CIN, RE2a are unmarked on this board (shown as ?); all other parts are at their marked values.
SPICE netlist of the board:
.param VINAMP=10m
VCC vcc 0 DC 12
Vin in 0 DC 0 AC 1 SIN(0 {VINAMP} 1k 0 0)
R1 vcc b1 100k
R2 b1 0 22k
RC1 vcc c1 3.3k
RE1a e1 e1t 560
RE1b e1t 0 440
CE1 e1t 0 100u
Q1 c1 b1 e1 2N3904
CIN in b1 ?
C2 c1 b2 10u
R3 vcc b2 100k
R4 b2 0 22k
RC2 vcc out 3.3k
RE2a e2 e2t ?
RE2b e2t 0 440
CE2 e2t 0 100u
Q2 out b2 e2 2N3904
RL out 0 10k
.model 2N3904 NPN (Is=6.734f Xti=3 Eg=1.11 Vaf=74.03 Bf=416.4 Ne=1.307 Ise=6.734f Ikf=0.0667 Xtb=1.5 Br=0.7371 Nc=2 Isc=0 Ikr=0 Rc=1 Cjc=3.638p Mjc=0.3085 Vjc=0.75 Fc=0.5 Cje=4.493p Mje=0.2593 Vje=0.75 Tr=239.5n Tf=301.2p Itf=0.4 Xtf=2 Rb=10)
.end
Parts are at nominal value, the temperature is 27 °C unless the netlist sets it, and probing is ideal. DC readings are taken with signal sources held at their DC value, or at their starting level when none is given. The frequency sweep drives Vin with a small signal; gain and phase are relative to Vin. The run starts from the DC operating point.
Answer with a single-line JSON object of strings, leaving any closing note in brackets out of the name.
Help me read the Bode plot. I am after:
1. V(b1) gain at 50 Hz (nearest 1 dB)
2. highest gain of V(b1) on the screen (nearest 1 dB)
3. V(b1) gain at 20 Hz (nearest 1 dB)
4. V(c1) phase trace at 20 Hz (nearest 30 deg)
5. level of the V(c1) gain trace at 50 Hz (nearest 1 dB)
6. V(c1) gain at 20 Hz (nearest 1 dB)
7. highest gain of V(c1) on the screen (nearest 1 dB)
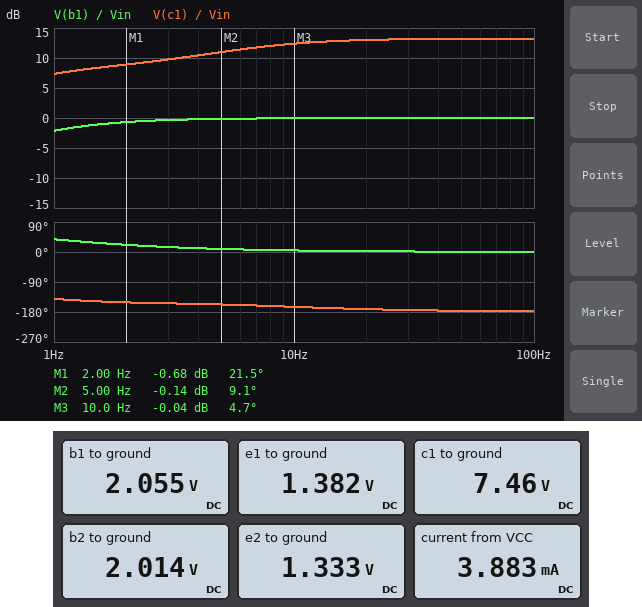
{"V(b1) gain at 50 Hz": "0 dB", "highest gain of V(b1) on the screen": "0 dB", "V(b1) gain at 20 Hz": "0 dB", "V(c1) phase trace at 20 Hz": "-180 deg", "level of the V(c1) gain trace at 50 Hz": "13 dB", "V(c1) gain at 20 Hz": "13 dB", "highest gain of V(c1) on the screen": "13 dB"}
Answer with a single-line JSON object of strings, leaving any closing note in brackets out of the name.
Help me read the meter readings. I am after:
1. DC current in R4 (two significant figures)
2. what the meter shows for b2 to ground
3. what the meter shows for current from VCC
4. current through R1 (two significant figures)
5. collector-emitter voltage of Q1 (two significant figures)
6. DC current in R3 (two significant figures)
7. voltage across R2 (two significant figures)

{"DC current in R4": "92 µA", "what the meter shows for b2 to ground": "2.014 V", "what the meter shows for current from VCC": "3.883 mA", "current through R1": "99 µA", "collector-emitter voltage of Q1": "6.1 V", "DC current in R3": "100 µA", "voltage across R2": "2.1 V"}
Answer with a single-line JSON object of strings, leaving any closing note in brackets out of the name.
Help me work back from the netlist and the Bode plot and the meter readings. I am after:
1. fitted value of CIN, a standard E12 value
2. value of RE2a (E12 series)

{"fitted value of CIN, a standard E12 value": "12 µF", "value of RE2a": "270 Ω"}
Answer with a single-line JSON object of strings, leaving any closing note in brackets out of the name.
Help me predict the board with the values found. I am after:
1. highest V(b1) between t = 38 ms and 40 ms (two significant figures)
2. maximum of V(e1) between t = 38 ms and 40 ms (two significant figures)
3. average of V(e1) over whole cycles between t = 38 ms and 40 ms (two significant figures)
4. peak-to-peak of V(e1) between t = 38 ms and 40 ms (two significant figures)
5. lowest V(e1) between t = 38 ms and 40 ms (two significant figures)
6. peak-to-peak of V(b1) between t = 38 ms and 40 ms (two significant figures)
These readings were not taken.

{"highest V(b1) between t = 38 ms and 40 ms": "2.1 V", "maximum of V(e1) between t = 38 ms and 40 ms": "1.4 V", "average of V(e1) over whole cycles between t = 38 ms and 40 ms": "1.4 V", "peak-to-peak of V(e1) between t = 38 ms and 40 ms": "19 mV", "lowest V(e1) between t = 38 ms and 40 ms": "1.4 V", "peak-to-peak of V(b1) between t = 38 ms and 40 ms": "20 mV"}
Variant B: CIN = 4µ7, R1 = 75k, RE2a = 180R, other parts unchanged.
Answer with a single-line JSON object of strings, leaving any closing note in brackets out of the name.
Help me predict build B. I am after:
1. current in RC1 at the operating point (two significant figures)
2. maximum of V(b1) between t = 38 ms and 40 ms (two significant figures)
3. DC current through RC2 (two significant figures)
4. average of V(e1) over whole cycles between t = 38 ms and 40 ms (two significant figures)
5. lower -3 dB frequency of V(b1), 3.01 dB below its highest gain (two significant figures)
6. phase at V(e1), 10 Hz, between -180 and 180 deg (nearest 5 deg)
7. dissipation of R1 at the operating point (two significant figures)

{"current in RC1 at the operating point": "1.9 mA", "maximum of V(b1) between t = 38 ms and 40 ms": "2.6 V", "DC current through RC2": "2.5 mA", "average of V(e1) over whole cycles between t = 38 ms and 40 ms": "1.9 V", "lower -3 dB frequency of V(b1), 3.01 dB below its highest gain": "2.2 Hz", "phase at V(e1), 10 Hz, between -180 and 180 deg": "10 deg", "dissipation of R1 at the operating point": "1.2 mW"}
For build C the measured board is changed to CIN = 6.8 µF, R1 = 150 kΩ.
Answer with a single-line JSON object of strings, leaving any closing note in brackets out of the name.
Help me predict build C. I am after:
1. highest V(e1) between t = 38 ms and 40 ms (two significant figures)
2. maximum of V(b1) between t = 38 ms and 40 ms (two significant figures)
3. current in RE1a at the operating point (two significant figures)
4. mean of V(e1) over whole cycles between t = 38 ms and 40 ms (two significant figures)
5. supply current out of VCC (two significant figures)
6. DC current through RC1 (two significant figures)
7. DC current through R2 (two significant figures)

{"highest V(e1) between t = 38 ms and 40 ms": "820 mV", "maximum of V(b1) between t = 38 ms and 40 ms": "1.5 V", "current in RE1a at the operating point": "810 µA", "mean of V(e1) over whole cycles between t = 38 ms and 40 ms": "810 mV", "supply current out of VCC": "3.3 mA", "DC current through RC1": "800 µA", "DC current through R2": "67 µA"}
